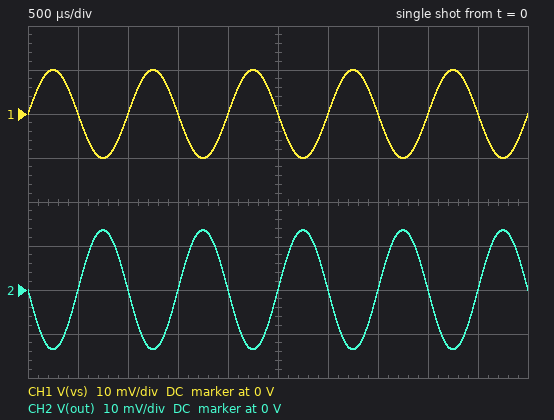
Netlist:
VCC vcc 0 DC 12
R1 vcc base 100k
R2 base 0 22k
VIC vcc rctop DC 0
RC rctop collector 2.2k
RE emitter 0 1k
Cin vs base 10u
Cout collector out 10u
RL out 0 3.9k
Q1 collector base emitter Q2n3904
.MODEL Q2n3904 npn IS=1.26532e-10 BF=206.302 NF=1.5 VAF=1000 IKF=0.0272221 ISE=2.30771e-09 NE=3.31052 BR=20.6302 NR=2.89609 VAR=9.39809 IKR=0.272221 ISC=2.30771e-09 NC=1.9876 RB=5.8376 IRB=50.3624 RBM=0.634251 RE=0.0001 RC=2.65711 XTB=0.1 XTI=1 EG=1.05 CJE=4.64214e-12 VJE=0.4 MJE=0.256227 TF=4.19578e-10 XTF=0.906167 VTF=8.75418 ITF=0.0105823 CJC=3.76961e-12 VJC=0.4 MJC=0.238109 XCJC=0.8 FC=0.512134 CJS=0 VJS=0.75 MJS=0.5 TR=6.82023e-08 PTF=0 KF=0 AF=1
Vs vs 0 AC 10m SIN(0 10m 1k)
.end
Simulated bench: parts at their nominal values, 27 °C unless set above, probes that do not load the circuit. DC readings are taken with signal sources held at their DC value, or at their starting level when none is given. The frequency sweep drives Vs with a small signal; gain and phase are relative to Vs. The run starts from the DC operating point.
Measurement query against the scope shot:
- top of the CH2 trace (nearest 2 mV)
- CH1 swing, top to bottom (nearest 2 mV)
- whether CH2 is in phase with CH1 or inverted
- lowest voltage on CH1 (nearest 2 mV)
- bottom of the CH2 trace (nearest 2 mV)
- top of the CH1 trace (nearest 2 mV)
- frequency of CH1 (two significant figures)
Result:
14 mV
20 mV
inverted
-10 mV
-14 mV
10 mV
1.0 kHz
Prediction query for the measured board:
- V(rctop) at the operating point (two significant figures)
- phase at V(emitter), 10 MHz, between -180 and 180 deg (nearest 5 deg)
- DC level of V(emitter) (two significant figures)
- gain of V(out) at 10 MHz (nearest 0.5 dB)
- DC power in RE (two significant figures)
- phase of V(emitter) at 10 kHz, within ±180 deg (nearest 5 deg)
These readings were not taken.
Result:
12 V
0 deg
1.3 V
2.5 dB
1.8 mW
0 deg
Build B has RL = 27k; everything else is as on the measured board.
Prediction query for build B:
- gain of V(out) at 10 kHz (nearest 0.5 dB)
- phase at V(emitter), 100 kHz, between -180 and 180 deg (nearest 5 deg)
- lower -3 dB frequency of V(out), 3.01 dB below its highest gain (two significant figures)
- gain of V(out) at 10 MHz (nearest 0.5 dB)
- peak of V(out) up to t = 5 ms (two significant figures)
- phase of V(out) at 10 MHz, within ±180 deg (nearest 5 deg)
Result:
6.0 dB
0 deg
1.2 Hz
5.5 dB
20 mV
155 deg
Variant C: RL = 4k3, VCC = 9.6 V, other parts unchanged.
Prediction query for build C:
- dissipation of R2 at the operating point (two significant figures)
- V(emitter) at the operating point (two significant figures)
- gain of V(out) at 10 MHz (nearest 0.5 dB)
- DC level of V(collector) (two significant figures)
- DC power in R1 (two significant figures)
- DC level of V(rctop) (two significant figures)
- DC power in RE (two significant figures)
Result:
110 µW
960 mV
3.0 dB
7.5 V
640 µW
9.6 V
930 µW
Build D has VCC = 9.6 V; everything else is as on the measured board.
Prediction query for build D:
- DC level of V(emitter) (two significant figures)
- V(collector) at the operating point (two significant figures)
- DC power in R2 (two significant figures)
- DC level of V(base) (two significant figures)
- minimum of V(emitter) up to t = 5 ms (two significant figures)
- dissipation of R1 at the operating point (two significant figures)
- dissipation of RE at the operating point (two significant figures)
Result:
960 mV
7.5 V
110 µW
1.6 V
950 mV
640 µW
930 µW
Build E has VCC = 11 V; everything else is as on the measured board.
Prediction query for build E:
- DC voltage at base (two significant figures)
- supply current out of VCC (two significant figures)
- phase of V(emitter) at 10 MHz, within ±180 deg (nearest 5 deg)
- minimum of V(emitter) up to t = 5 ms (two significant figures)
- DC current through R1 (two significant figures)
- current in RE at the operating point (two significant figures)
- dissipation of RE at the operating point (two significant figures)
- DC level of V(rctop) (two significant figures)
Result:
1.8 V
1.3 mA
0 deg
1.2 V
92 µA
1.2 mA
1.4 mW
11 V
